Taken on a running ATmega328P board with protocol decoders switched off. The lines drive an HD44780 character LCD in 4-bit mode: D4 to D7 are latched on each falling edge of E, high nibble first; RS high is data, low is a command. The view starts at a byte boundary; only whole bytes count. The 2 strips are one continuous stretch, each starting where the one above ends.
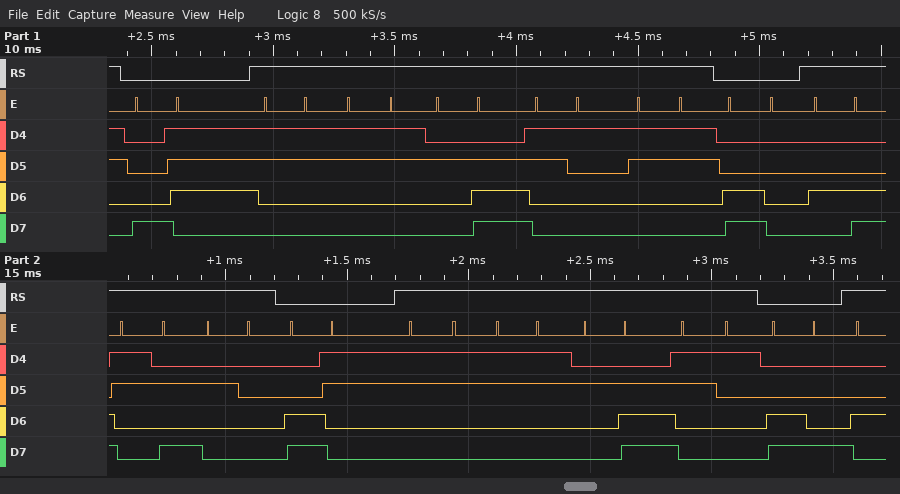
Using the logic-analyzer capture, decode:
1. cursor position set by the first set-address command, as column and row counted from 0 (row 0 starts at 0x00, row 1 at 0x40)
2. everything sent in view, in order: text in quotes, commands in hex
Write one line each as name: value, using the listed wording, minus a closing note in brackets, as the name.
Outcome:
cursor position set by the first set-address command, as column and row counted from 0: column 7, row 0
everything sent in view, in order: text in quotes, commands in hex: 0x87 "33.13" 0xC0 "L: " 0xC3 "33.1" 0xC8
